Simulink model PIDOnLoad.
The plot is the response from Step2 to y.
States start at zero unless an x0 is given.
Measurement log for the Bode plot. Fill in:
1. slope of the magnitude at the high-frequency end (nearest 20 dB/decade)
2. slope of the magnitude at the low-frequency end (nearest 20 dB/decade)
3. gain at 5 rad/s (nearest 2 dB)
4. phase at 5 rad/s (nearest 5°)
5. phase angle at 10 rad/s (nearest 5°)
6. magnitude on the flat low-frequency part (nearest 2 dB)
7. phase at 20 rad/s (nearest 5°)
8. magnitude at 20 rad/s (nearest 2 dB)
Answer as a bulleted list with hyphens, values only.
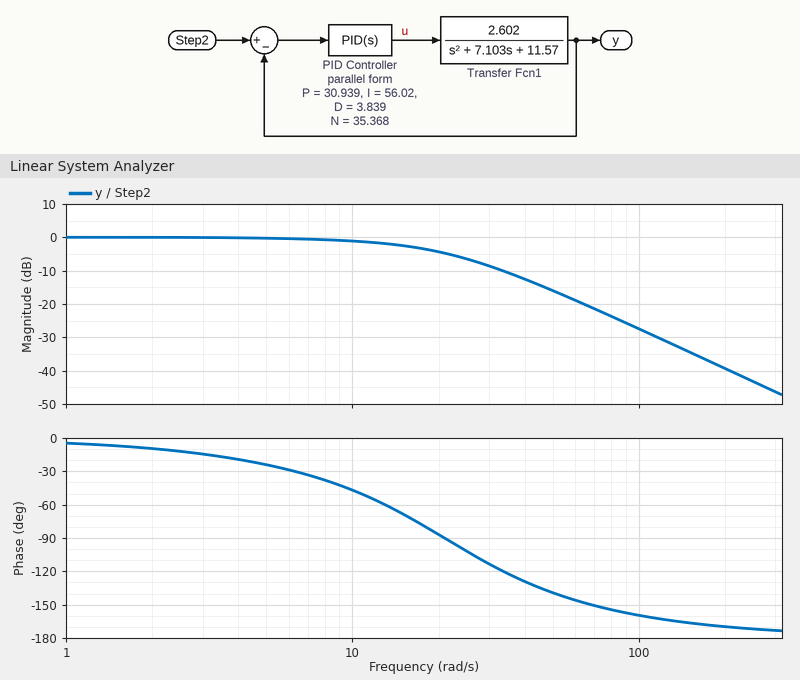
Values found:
- -40 dB/decade
- 0 dB/decade
- 0 dB
- -25°
- -45°
- 0 dB
- -85°
- -4 dB
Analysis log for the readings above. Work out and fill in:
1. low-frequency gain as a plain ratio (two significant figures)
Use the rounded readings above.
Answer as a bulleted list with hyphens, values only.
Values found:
- 1.0
